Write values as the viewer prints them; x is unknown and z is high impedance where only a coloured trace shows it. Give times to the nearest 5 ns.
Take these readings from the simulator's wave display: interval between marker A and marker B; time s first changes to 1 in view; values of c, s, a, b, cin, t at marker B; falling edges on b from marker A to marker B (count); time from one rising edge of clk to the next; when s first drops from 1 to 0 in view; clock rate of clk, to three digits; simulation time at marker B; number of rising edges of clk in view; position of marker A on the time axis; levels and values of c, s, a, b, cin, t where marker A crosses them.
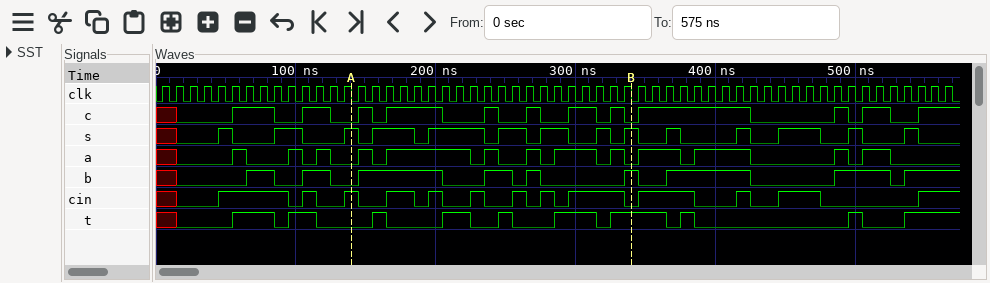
200 ns
45 ns
c=0, s=1, a=0, b=1, cin=0, t=1
3
10 ns
55 ns
100 MHz
340 ns
57
140 ns
c=0, s=1, a=0, b=0, cin=1, t=0
